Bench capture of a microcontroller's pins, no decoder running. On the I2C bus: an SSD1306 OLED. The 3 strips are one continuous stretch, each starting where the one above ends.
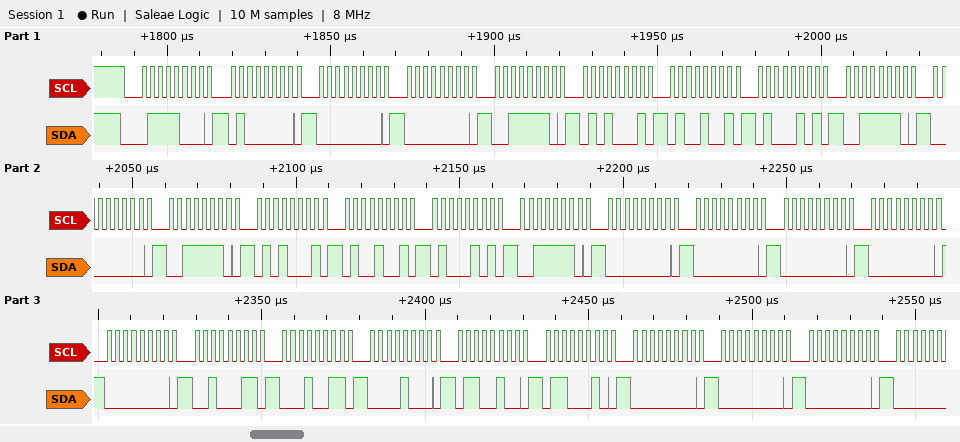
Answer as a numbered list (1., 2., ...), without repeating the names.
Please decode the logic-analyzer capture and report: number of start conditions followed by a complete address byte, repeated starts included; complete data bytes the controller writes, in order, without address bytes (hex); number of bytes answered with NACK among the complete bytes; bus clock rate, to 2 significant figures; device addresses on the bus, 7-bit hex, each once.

1. 1
2. 40 00 00 3E 51 49 45 3E 00 3E 51 49 45 3E 00 00 00 00 00 23 13 08 64 62 00 00 00
3. 0
4. 400 kHz
5. 0x3C
